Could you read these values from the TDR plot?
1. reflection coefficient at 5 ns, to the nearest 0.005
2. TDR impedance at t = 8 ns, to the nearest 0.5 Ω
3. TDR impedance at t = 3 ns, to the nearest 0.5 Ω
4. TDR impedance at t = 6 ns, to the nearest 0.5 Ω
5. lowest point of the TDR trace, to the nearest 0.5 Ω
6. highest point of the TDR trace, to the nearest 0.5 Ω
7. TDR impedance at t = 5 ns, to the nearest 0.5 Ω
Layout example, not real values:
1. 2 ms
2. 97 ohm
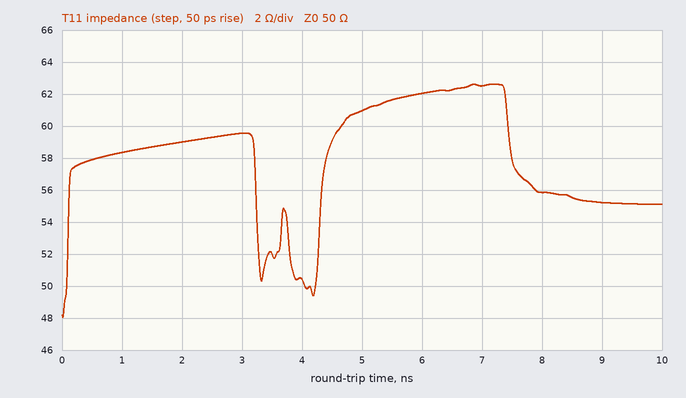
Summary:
1. +0.100
2. 56.0 Ω
3. 59.5 Ω
4. 62.0 Ω
5. 48.0 Ω
6. 62.5 Ω
7. 61.0 Ω
